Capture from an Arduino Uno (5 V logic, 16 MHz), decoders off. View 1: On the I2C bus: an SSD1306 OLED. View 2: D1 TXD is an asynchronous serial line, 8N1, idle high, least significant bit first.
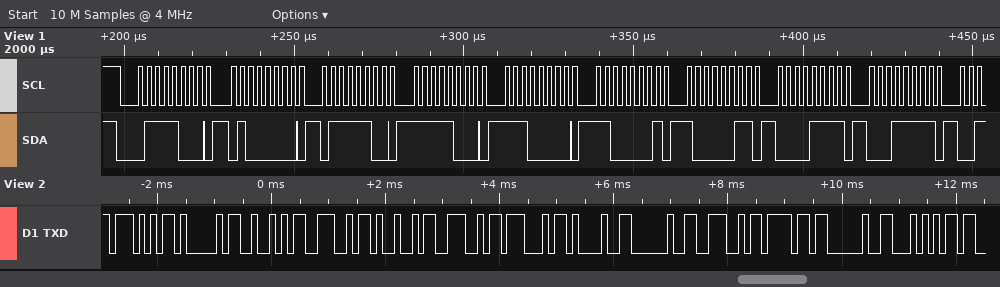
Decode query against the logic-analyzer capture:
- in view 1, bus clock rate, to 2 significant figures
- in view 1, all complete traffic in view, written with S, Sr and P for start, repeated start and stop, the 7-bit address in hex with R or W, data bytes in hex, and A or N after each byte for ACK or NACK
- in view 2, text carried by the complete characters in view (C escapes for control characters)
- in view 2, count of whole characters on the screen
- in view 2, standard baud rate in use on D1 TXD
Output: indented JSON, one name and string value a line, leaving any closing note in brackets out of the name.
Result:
{
  "in view 1, bus clock rate, to 2 significant figures": "400 kHz",
  "in view 1, all complete traffic in view, written with S, Sr and P for start, repeated start and stop, the 7-bit address in hex with R or W, data bytes in hex, and A or N after each byte for ACK or NACK": "S 3CW A 40 A 7C A F8 A E0 A C1 A 83 A 0F A 1F A",
  "in view 2, text carried by the complete characters in view": "\"WARNING! No T\"",
  "in view 2, count of whole characters on the screen": "13",
  "in view 2, standard baud rate in use on D1 TXD": "9600 baud"
}
